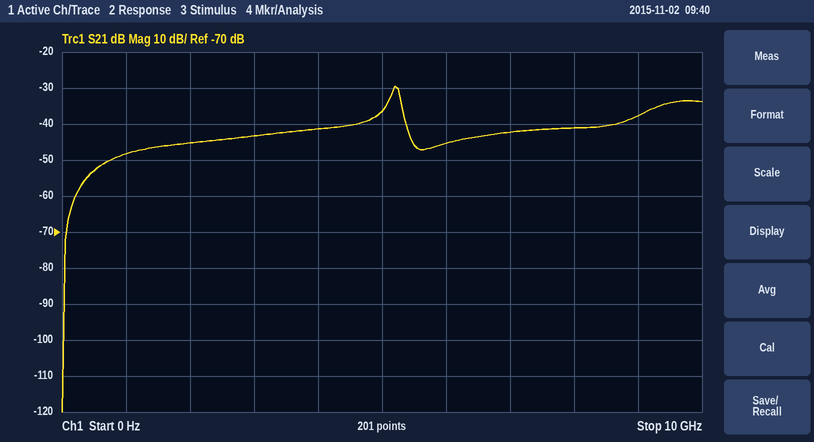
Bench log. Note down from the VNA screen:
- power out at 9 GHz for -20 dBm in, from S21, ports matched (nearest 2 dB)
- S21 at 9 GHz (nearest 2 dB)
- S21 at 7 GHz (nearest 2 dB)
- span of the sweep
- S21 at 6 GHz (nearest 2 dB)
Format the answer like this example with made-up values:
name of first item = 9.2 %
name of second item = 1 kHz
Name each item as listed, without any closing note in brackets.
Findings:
power out at 9 GHz for -20 dBm in, from S21, ports matched = -58 dBm
S21 at 9 GHz = -38 dB
S21 at 7 GHz = -42 dB
span of the sweep = 10 GHz
S21 at 6 GHz = -46 dB
